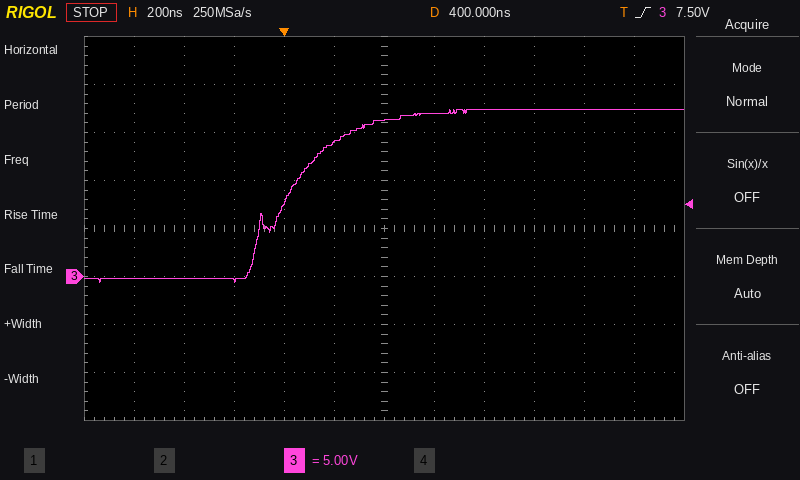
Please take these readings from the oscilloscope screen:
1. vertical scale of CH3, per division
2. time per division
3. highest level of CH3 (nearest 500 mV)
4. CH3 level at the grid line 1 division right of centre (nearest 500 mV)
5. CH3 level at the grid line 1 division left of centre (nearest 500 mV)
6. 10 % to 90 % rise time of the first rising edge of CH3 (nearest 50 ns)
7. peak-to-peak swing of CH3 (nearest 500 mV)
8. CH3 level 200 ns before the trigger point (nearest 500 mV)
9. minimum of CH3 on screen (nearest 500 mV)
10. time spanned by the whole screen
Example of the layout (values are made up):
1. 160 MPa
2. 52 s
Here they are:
1. 5 V
2. 200 ns
3. 17.5 V
4. 17.0 V
5. 14.0 V
6. 450 ns
7. 18.0 V
8. -500 mV
9. -500 mV
10. 2.4 µs
